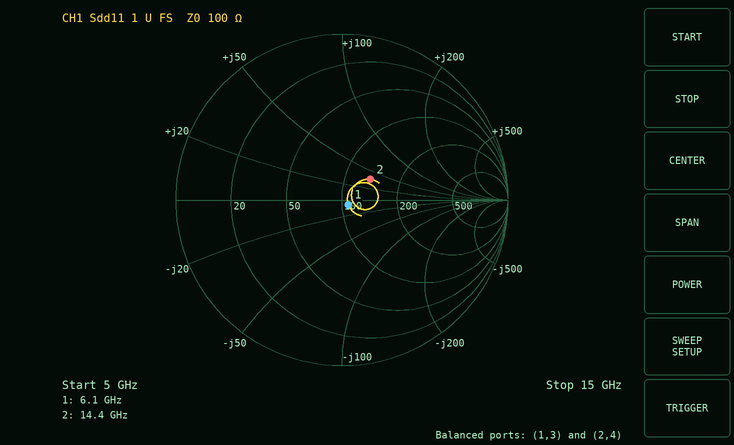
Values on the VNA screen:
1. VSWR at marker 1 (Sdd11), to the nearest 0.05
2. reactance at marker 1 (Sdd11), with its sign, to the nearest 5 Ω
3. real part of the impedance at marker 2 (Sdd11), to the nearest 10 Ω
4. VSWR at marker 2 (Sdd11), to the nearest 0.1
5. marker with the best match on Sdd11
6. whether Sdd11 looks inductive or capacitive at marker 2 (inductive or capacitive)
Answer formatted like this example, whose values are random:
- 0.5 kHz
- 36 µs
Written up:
- 1.10
- -5 Ω
- 140 Ω
- 1.5
- marker 1
- inductive
